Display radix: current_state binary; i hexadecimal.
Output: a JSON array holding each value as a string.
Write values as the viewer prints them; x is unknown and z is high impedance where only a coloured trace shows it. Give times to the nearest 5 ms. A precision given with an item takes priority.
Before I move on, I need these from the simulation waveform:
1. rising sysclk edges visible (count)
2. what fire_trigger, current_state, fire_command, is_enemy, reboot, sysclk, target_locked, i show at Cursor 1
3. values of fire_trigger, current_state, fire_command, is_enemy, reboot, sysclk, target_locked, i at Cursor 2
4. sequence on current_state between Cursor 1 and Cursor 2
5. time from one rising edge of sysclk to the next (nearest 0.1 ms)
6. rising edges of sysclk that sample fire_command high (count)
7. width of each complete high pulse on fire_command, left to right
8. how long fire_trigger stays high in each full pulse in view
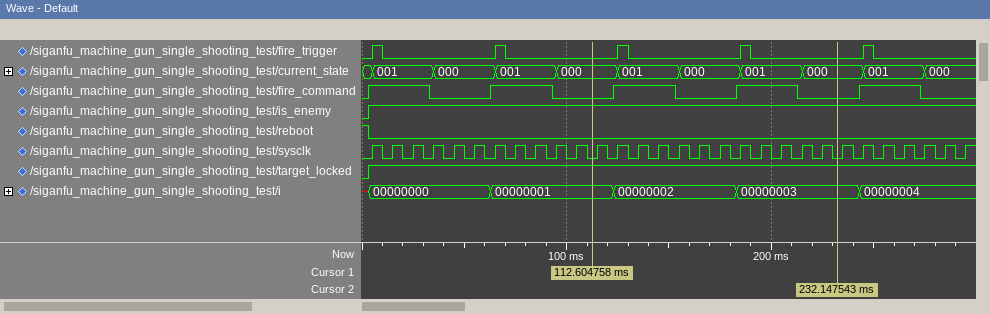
["30", "fire_trigger=0, current_state=000, fire_command=0, is_enemy=1, reboot=0, sysclk=0, target_locked=1, i=00000001", "fire_trigger=0, current_state=000, fire_command=0, is_enemy=1, reboot=0, sysclk=0, target_locked=1, i=00000003", "000, 001, 000, 001, 000", "10 ms", "15", "30 ms, 30 ms, 30 ms, 30 ms, 30 ms", "5 ms, 5 ms, 5 ms, 5 ms, 5 ms"]
